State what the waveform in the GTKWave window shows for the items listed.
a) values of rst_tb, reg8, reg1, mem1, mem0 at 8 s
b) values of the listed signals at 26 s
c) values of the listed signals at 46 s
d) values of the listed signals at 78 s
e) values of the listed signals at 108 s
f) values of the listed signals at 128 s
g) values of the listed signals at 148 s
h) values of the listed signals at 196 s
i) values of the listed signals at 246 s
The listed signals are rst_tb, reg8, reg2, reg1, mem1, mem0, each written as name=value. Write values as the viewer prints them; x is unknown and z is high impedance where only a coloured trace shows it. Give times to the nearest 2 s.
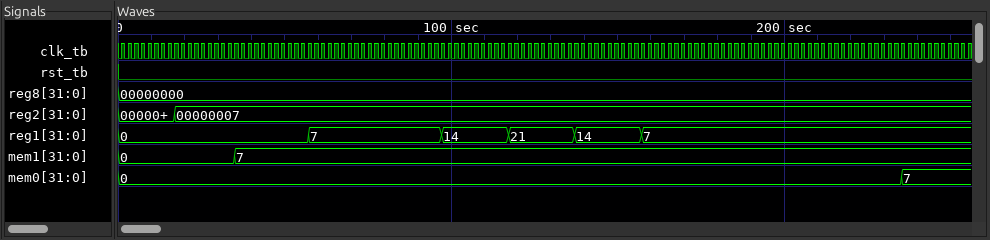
rst_tb=0, reg8=00000000, reg1=0, mem1=0, mem0=0
rst_tb=0, reg8=00000000, reg2=00000007, reg1=0, mem1=0, mem0=0
rst_tb=0, reg8=00000000, reg2=00000007, reg1=0, mem1=7, mem0=0
rst_tb=0, reg8=00000000, reg2=00000007, reg1=7, mem1=7, mem0=0
rst_tb=0, reg8=00000000, reg2=00000007, reg1=14, mem1=7, mem0=0
rst_tb=0, reg8=00000000, reg2=00000007, reg1=21, mem1=7, mem0=0
rst_tb=0, reg8=00000000, reg2=00000007, reg1=14, mem1=7, mem0=0
rst_tb=0, reg8=00000000, reg2=00000007, reg1=7, mem1=7, mem0=0
rst_tb=0, reg8=00000000, reg2=00000007, reg1=7, mem1=7, mem0=7
